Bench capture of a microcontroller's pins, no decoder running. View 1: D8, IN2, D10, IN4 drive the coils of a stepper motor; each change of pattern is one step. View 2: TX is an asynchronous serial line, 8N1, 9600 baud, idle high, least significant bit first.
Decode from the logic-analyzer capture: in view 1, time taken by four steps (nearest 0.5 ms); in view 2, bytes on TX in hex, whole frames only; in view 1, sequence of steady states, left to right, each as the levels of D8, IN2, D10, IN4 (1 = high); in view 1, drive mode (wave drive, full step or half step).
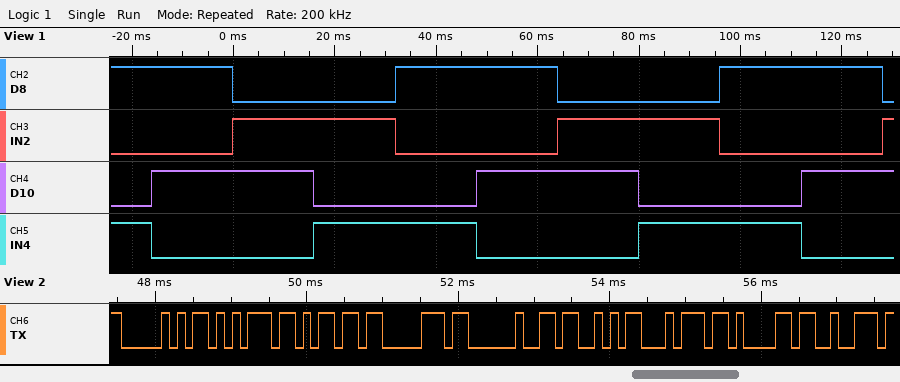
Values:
64.0 ms
50 75 6D 70 20 53 74 61 72
1001 1010 0110 0101 1001 1010 0110 0101 1001 1010 0110
full step
